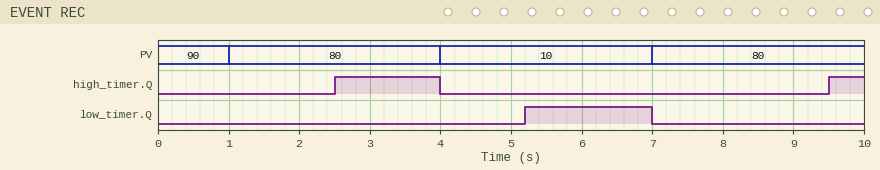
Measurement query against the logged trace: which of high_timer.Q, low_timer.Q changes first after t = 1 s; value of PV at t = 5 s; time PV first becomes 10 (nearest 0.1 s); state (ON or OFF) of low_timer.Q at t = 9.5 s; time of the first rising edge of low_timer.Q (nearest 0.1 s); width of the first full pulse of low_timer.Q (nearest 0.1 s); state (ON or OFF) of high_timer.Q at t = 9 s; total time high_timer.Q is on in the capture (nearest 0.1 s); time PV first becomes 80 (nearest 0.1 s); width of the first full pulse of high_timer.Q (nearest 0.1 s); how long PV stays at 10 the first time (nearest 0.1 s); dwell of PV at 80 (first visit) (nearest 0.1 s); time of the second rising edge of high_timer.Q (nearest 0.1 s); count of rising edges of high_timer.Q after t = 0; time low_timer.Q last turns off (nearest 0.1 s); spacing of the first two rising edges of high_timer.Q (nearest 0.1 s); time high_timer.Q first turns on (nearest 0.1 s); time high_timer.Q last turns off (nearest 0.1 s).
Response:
high_timer.Q
10
4.0 s
OFF
5.2 s
1.8 s
OFF
2.0 s
1.0 s
1.5 s
3.0 s
3.0 s
9.5 s
2
7.0 s
7.0 s
2.5 s
4.0 s
